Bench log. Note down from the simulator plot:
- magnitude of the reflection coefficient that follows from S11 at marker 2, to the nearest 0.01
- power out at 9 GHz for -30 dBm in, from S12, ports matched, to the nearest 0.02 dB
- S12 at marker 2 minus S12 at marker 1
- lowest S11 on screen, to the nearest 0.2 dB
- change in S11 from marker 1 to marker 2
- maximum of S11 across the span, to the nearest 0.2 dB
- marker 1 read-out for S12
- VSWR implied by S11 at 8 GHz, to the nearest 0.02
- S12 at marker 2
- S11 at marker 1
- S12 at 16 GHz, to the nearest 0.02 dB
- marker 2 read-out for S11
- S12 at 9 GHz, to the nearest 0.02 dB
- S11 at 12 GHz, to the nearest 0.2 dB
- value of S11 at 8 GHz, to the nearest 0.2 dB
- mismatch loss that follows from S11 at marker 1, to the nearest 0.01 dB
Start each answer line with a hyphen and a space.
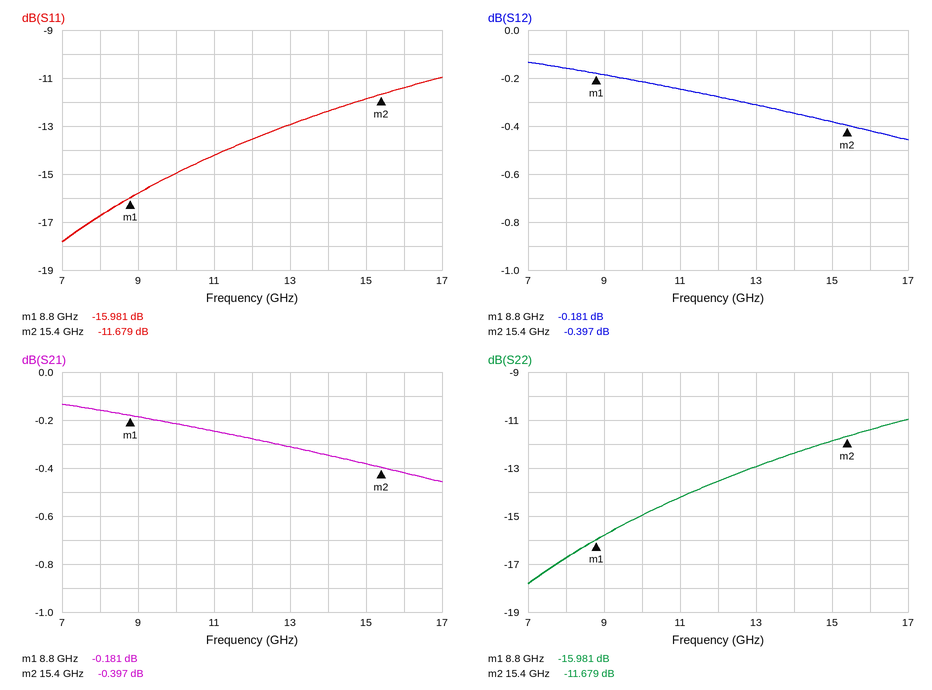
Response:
- 0.26
- -30.18 dBm
- -0.216 dB
- -17.8 dB
- 4.302 dB
- -11.0 dB
- -0.181 dB
- 1.34
- -0.397 dB
- -15.981 dB
- -0.42 dB
- -11.679 dB
- -0.18 dB
- -13.6 dB
- -16.8 dB
- 0.11 dB
